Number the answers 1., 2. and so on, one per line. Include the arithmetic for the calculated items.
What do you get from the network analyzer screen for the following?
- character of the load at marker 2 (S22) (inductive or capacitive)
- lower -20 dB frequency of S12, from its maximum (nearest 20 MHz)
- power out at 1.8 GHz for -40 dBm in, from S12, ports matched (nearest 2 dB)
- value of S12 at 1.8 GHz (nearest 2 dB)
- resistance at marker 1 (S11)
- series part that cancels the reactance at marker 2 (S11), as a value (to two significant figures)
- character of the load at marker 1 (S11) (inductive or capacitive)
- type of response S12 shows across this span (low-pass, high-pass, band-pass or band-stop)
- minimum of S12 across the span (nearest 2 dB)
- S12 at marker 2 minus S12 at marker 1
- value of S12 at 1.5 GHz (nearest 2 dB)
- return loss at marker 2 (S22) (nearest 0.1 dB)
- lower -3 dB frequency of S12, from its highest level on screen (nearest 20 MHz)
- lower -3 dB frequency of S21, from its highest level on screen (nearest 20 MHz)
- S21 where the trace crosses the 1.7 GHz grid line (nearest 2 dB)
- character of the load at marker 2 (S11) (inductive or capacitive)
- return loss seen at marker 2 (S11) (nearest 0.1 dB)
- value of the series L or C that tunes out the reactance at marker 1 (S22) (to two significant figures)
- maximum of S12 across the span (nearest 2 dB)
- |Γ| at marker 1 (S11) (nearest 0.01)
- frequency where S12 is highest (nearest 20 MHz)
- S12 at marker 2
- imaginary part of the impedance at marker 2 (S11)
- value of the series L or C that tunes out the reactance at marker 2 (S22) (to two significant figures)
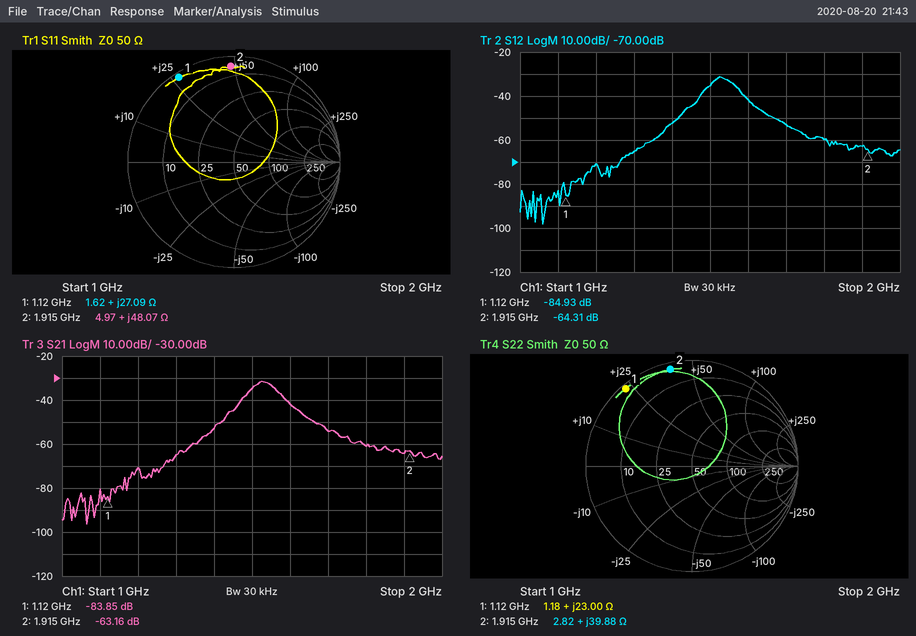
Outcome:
1. inductive
2. 1.40 GHz
3. -40 dBm + (-60 dB) = -100 dBm
4. -60 dB
5. 1.62 Ω
6. C = 1/(2π × 1.915 GHz × 48.07 Ω) ≈ 1.7 pF
7. inductive
8. band-pass
9. -98 dB
10. -64.31 − (-84.93) = 20.62 dB
11. -36 dB
12. 0.6 dB
13. 1.50 GHz
14. 1.50 GHz
15. -54 dB
16. inductive
17. 0.9 dB
18. C = 1/(2π × 1.12 GHz × 23 Ω) ≈ 6.2 pF
19. -32 dB
20. 0.95
21. 1.52 GHz
22. -64.31 dB
23. +48.07 Ω
24. C = 1/(2π × 1.915 GHz × 39.88 Ω) ≈ 2.1 pF
